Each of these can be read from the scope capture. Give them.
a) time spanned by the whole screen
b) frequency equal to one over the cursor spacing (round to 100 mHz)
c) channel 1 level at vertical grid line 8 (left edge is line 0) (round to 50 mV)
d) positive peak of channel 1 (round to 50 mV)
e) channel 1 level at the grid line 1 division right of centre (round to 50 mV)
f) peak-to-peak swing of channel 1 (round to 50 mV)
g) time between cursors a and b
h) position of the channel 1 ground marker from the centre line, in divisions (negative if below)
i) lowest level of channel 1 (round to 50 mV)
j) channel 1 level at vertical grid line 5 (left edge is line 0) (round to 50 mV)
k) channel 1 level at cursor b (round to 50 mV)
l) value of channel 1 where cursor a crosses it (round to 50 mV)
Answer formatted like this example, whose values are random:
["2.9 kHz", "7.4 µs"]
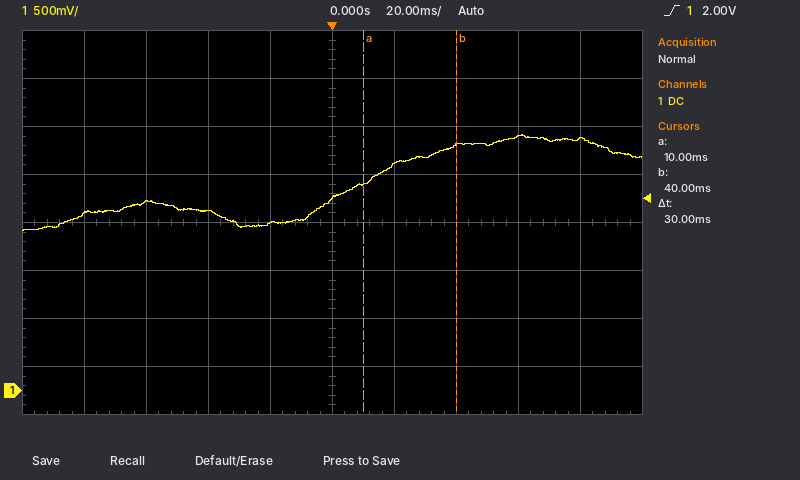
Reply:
["200 ms", "33.3 Hz", "2.65 V", "2.65 V", "2.35 V", "1.00 V", "30 ms", "-3.5 div", "1.65 V", "2.00 V", "2.55 V", "2.15 V"]
